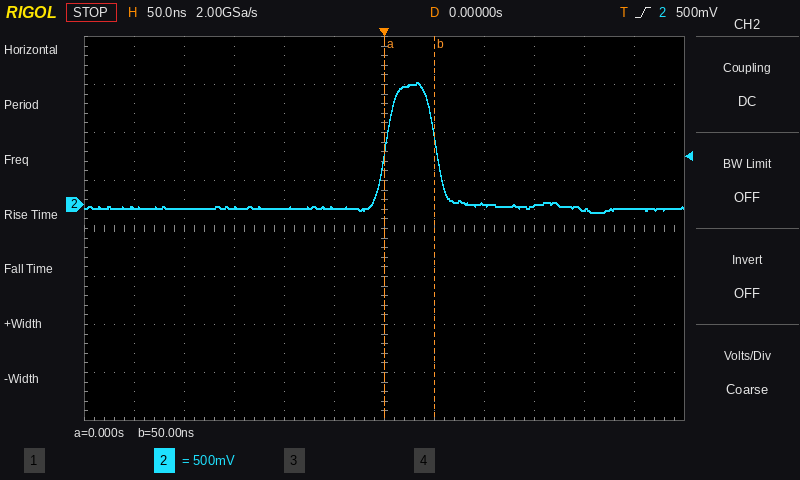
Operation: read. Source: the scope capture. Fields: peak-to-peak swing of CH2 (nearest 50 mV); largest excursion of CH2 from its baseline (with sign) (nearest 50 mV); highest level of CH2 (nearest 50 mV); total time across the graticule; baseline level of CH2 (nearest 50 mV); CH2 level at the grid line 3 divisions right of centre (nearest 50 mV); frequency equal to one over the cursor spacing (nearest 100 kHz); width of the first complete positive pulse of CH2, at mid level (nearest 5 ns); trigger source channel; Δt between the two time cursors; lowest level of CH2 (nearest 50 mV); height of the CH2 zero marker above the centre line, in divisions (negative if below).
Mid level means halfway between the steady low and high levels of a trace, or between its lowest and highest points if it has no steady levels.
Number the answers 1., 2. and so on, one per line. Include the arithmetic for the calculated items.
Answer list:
1. 1.25 V − (-100 mV) = 1.35 V
2. 1.25 V − (-50 mV) = +1.30 V
3. 1.25 V
4. 600 ns
5. -50 mV
6. 0 mV
7. 1 / 50 ns ≈ 20.0 MHz
8. 50 ns
9. CH2
10. 50 ns − (0 s) = 50 ns
11. -100 mV
12. +0.5 div
